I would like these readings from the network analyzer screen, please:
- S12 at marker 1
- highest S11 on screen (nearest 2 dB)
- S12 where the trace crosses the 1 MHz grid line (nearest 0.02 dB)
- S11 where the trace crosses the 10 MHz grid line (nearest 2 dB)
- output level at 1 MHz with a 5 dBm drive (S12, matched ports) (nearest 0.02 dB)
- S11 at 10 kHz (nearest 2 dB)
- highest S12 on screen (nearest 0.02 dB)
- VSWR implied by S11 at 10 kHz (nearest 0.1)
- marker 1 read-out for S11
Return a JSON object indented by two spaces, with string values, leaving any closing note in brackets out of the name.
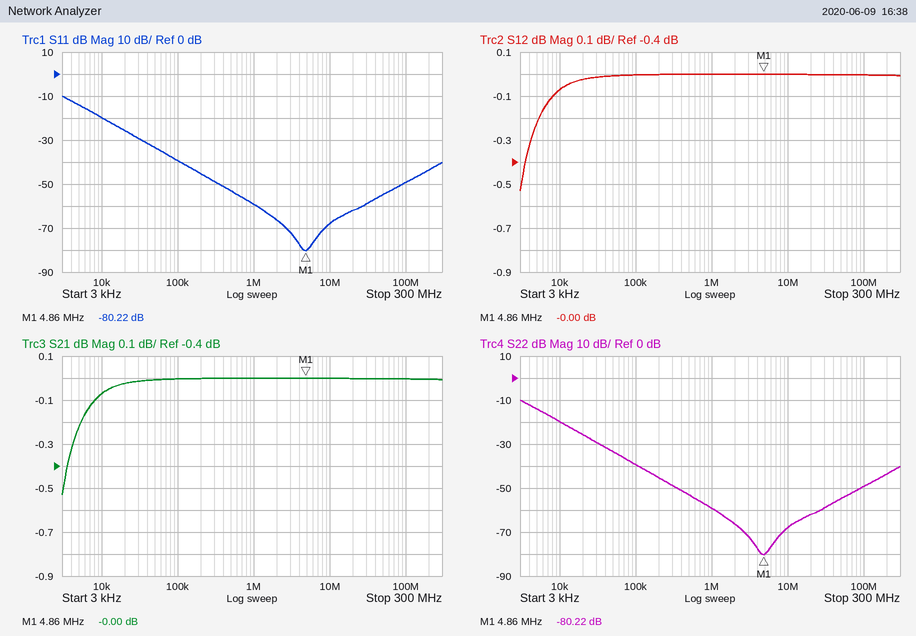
{
  "S12 at marker 1": "-0.00 dB",
  "highest S11 on screen": "-10 dB",
  "S12 where the trace crosses the 1 MHz grid line": "0.00 dB",
  "S11 where the trace crosses the 10 MHz grid line": "-68 dB",
  "output level at 1 MHz with a 5 dBm drive (S12, matched ports)": "5.00 dBm",
  "S11 at 10 kHz": "-20 dB",
  "highest S12 on screen": "0.00 dB",
  "VSWR implied by S11 at 10 kHz": "1.2",
  "marker 1 read-out for S11": "-80.22 dB"
}
